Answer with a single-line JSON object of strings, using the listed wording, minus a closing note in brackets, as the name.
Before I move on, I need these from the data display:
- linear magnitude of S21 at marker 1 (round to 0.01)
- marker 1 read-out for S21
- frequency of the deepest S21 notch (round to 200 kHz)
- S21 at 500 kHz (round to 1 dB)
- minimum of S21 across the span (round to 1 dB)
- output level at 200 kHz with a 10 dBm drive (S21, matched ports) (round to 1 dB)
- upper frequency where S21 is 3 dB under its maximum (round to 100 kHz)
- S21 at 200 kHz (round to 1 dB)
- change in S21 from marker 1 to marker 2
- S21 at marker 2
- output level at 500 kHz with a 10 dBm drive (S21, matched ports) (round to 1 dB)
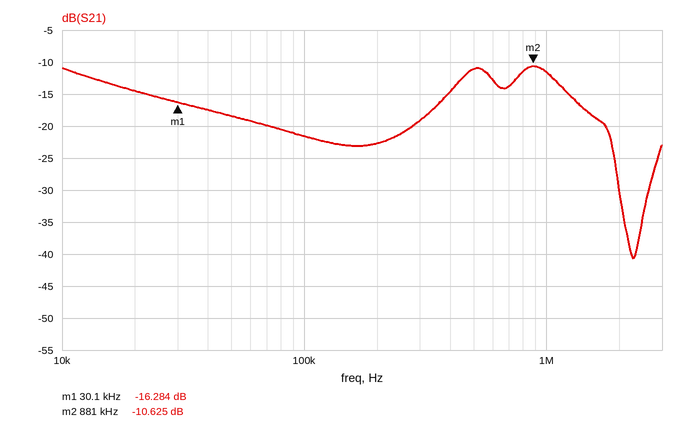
{"linear magnitude of S21 at marker 1": "0.15", "marker 1 read-out for S21": "-16.284 dB", "frequency of the deepest S21 notch": "2.2 MHz", "S21 at 500 kHz": "-11 dB", "minimum of S21 across the span": "-41 dB", "output level at 200 kHz with a 10 dBm drive (S21, matched ports)": "-13 dBm", "upper frequency where S21 is 3 dB under its maximum": "1.1 MHz", "S21 at 200 kHz": "-23 dB", "change in S21 from marker 1 to marker 2": "5.659 dB", "S21 at marker 2": "-10.625 dB", "output level at 500 kHz with a 10 dBm drive (S21, matched ports)": "-1 dBm"}
